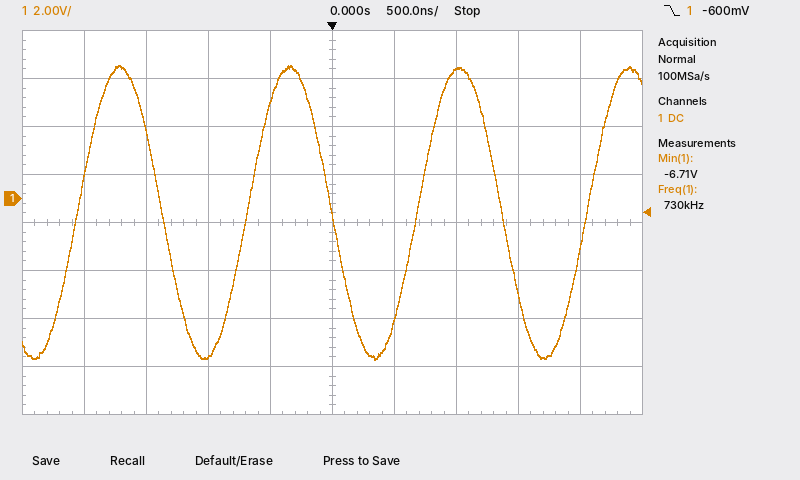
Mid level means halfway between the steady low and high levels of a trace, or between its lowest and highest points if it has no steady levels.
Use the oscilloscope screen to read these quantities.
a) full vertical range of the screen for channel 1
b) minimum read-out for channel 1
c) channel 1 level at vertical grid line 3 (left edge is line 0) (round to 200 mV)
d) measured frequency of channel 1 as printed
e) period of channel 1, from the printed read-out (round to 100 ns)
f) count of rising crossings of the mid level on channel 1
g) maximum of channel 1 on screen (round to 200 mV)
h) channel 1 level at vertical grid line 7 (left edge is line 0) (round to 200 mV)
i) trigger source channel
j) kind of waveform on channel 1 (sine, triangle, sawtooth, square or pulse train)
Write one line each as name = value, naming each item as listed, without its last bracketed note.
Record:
full vertical range of the screen for channel 1 = 16 V
minimum read-out for channel 1 = -6.71 V
channel 1 level at vertical grid line 3 (left edge is line 0) = -6.6 V
measured frequency of channel 1 as printed = 730 kHz
period of channel 1, from the printed read-out = 1.4 µs
count of rising crossings of the mid level on channel 1 = 4
maximum of channel 1 on screen = 5.6 V
channel 1 level at vertical grid line 7 (left edge is line 0) = 5.4 V
trigger source channel = channel 1
kind of waveform on channel 1 = sine
